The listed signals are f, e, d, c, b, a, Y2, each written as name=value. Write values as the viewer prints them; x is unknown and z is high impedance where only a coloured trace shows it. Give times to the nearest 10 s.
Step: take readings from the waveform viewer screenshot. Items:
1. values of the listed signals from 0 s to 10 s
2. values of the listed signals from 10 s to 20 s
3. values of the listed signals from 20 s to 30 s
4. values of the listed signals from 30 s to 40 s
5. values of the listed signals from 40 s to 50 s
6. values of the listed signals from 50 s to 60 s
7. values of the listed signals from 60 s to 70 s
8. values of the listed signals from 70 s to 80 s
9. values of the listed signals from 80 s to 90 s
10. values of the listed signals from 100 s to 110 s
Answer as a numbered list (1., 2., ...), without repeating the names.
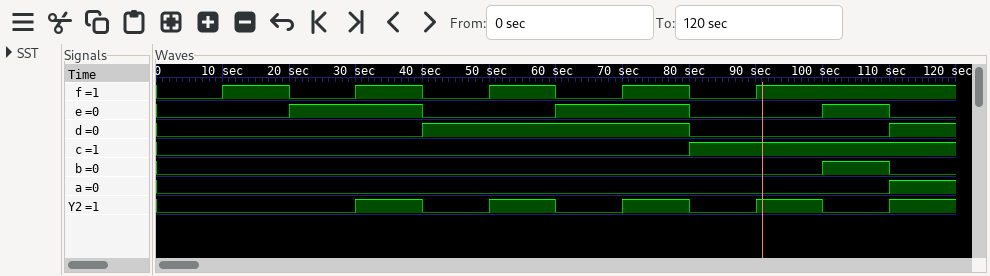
1. f=0, e=0, d=0, c=0, b=0, a=0, Y2=0
2. f=1, e=0, d=0, c=0, b=0, a=0, Y2=0
3. f=0, e=1, d=0, c=0, b=0, a=0, Y2=0
4. f=1, e=1, d=0, c=0, b=0, a=0, Y2=1
5. f=0, e=0, d=1, c=0, b=0, a=0, Y2=0
6. f=1, e=0, d=1, c=0, b=0, a=0, Y2=1
7. f=0, e=1, d=1, c=0, b=0, a=0, Y2=0
8. f=1, e=1, d=1, c=0, b=0, a=0, Y2=1
9. f=0, e=0, d=0, c=1, b=0, a=0, Y2=0
10. f=1, e=1, d=0, c=1, b=1, a=0, Y2=0
